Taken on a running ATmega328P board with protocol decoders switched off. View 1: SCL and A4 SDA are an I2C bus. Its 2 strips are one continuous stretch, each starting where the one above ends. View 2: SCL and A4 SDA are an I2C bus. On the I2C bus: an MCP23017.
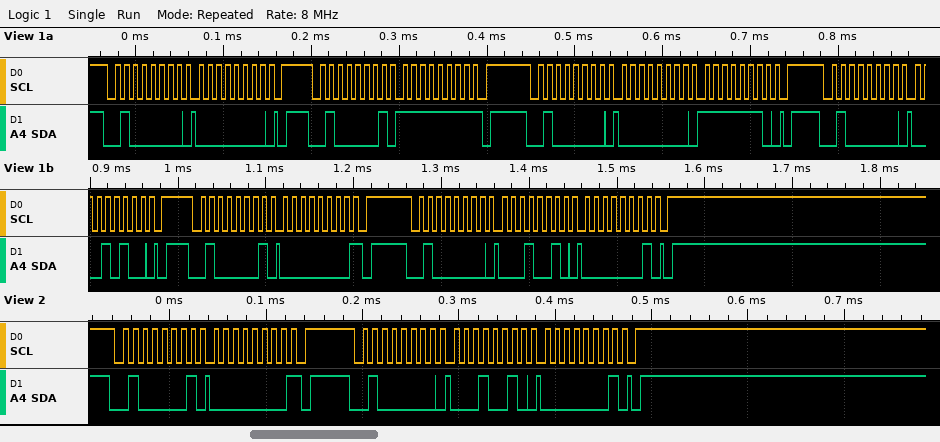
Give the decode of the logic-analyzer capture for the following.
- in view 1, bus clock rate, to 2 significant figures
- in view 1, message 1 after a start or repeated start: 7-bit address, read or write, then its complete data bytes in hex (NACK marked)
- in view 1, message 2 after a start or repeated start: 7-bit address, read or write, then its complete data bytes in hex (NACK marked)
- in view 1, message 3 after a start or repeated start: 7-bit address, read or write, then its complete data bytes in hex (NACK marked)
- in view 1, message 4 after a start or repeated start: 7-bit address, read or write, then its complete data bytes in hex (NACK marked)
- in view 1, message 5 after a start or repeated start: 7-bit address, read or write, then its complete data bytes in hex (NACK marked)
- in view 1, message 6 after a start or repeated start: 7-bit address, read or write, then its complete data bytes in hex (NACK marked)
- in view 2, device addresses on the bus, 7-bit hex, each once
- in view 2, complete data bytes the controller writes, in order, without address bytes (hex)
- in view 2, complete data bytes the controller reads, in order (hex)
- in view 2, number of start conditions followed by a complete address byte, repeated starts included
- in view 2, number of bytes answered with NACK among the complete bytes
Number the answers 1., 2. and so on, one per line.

1. 100 kHz
2. 0x20 write: 00
3. 0x20 read: FF NACK
4. 0x20 write: 00 FE
5. 0x20 write: 14
6. 0x20 read: 00 NACK
7. 0x20 write: 12 01
8. 0x20
9. 12 01
10. 00
11. 2
12. 1
